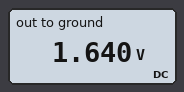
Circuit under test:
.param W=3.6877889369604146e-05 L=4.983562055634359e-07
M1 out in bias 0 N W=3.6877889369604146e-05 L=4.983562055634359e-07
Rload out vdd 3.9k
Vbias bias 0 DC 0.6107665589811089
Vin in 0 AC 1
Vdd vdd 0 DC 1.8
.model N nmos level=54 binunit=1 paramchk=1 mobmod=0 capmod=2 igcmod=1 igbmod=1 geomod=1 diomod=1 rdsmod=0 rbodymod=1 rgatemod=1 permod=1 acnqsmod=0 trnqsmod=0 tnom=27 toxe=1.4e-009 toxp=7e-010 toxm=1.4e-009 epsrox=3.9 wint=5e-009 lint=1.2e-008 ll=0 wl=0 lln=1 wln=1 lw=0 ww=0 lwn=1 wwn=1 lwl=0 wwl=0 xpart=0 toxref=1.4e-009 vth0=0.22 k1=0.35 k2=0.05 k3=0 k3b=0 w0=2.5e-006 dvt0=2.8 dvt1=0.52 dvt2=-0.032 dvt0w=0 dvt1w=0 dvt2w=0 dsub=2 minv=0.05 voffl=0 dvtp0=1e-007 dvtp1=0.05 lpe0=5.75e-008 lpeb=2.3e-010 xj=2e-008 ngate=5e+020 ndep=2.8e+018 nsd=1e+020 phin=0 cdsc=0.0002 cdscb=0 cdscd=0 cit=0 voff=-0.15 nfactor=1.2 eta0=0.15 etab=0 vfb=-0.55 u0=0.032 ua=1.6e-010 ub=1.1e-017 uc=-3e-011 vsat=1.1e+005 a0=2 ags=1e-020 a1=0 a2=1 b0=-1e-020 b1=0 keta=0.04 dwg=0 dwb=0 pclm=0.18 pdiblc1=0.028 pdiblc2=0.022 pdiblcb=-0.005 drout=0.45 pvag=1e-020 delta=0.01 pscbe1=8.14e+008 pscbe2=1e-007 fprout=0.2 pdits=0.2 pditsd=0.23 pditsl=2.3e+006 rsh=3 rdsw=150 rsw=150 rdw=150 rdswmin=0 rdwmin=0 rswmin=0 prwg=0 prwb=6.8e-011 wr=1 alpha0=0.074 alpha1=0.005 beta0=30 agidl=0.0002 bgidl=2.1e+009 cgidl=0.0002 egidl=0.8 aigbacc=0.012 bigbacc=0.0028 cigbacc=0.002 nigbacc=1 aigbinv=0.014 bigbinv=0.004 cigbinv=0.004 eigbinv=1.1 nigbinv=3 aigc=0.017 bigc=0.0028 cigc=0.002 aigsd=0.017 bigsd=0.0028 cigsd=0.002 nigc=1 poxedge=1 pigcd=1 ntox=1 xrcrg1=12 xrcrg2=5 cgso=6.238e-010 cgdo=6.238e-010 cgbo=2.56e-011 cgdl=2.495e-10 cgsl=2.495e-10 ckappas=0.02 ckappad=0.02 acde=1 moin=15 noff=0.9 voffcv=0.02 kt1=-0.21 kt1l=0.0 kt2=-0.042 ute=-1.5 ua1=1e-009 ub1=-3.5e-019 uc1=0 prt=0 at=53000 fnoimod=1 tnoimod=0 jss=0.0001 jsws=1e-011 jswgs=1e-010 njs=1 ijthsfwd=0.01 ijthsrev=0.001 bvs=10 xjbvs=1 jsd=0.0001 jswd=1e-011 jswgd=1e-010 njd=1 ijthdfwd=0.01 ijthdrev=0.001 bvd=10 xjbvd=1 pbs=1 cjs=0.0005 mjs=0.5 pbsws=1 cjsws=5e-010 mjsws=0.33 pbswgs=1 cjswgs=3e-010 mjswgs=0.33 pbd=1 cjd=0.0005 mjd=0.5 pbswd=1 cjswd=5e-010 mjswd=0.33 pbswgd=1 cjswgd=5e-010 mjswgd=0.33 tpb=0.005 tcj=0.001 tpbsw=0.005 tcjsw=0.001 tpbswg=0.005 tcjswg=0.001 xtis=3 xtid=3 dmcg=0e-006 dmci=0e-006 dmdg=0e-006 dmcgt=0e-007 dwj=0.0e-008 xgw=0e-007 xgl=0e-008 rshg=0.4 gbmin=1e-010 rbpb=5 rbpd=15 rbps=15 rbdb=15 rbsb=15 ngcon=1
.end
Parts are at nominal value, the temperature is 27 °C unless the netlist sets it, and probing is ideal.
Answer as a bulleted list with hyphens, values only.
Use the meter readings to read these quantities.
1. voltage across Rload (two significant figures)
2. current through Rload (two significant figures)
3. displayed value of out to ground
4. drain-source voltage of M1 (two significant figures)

- 160 mV
- 41 µA
- 1.640 V
- 1.0 V
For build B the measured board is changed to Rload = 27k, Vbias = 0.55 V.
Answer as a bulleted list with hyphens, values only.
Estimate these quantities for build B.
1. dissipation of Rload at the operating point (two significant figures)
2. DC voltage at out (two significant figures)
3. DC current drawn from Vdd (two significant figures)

- 2.5 µW
- 1.5 V
- 9.5 µA
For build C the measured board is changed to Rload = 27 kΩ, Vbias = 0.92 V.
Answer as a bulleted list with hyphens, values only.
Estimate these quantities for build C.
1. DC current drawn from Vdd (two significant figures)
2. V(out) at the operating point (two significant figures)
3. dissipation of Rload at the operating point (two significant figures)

- 9.5 µA
- 1.5 V
- 2.5 µW
